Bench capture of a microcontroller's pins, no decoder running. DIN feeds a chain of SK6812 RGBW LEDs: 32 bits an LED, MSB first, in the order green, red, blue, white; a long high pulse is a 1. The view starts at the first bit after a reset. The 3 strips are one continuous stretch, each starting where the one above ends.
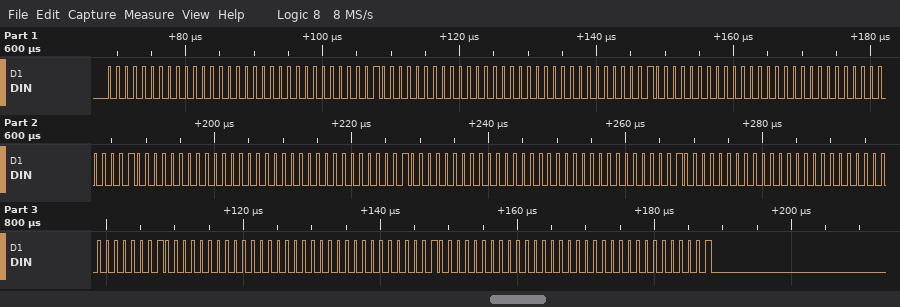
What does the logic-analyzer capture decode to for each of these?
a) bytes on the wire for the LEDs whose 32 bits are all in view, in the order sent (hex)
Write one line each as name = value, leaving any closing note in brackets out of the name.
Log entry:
bytes on the wire for the LEDs whose 32 bits are all in view, in the order sent = 00 00 00 01 00 00 00 01 00 00 00 01 00 00 00 01 00 00 00 01 00 00 00 01 00 00 00 01 00 00 00 01
